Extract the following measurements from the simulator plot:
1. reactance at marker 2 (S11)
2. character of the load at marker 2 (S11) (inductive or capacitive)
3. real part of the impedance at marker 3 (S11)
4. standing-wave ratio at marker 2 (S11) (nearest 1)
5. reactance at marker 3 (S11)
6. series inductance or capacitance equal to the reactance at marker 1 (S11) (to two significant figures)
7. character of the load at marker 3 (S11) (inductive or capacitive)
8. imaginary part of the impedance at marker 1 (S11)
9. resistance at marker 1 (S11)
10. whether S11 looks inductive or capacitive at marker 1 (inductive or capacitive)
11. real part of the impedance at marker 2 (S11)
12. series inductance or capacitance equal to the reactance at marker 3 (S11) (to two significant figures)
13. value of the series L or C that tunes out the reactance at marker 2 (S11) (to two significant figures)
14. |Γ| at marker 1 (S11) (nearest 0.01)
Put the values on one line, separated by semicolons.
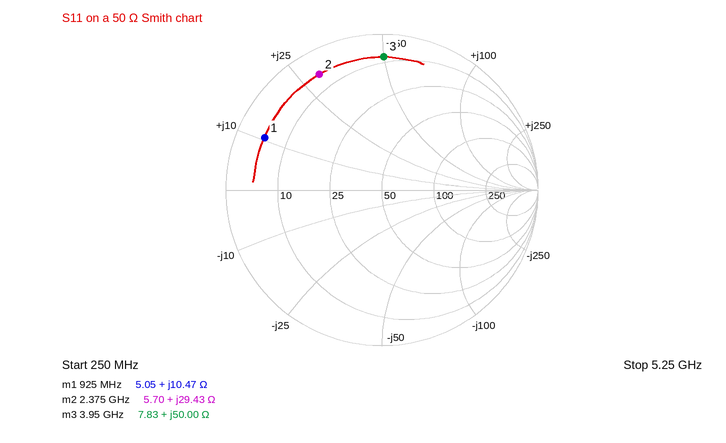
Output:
+29.43 Ω; inductive; 7.83 Ω; 12; +50.00 Ω; 1.8 nH; inductive; +10.47 Ω; 5.05 Ω; inductive; 5.70 Ω; 2.0 nH; 2.3 pF; 0.82
